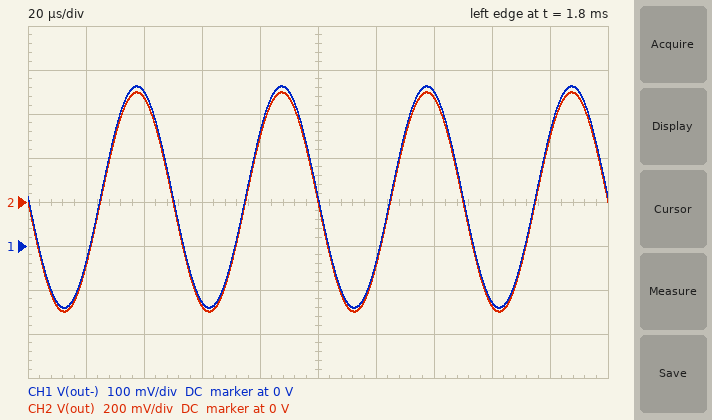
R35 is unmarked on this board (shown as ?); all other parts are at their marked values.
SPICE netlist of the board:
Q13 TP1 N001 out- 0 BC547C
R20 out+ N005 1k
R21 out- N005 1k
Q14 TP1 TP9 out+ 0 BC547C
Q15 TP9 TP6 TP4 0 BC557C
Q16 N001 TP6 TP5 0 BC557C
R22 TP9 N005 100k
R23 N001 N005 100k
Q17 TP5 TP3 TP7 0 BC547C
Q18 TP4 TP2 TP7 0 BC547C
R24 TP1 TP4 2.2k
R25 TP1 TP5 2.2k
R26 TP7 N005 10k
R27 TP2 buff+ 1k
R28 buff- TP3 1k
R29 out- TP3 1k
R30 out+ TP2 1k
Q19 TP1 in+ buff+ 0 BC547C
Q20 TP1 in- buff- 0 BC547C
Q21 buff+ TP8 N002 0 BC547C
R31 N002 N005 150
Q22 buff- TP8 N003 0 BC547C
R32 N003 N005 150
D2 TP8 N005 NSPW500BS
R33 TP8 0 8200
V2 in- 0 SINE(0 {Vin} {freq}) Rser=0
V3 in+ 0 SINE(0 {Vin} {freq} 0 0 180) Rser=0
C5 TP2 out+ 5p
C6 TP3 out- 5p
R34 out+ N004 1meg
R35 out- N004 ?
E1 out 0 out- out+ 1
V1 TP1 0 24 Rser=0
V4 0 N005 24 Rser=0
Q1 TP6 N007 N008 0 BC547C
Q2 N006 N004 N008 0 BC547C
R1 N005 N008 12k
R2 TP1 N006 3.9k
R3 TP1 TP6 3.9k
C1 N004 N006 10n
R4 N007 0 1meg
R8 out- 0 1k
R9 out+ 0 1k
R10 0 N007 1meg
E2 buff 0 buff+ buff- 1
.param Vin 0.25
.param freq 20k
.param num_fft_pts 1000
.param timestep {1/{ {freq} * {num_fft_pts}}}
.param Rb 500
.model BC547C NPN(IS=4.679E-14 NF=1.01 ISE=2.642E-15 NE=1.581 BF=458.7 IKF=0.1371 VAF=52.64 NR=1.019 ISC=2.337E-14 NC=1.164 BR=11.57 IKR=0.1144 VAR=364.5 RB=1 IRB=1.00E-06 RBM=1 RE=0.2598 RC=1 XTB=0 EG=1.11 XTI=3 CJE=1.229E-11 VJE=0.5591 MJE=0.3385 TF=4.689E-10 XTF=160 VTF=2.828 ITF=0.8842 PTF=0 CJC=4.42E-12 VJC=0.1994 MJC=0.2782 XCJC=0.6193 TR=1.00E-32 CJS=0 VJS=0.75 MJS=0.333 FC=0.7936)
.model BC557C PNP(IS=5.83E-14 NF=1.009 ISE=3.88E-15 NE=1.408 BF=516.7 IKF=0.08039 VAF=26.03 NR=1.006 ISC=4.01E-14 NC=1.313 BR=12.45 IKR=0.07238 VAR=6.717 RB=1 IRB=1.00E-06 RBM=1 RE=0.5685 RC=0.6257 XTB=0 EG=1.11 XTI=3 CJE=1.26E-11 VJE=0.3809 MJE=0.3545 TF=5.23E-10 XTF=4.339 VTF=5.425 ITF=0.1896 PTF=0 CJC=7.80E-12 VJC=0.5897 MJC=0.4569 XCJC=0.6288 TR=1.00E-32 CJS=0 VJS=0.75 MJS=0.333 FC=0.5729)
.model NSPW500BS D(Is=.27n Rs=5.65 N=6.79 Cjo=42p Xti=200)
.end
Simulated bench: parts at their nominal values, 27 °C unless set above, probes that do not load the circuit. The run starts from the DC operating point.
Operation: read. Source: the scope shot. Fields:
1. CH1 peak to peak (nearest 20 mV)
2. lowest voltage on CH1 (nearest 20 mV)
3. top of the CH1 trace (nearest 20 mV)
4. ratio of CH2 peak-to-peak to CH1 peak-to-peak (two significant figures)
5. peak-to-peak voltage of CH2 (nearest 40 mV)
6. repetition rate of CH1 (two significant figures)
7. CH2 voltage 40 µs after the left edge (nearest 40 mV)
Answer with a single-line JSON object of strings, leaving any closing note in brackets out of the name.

{"CH1 peak to peak": "500 mV", "lowest voltage on CH1": "-140 mV", "top of the CH1 trace": "360 mV", "ratio of CH2 peak-to-peak to CH1 peak-to-peak": "2.0", "peak-to-peak voltage of CH2": "1.00 V", "repetition rate of CH1": "20 kHz", "CH2 voltage 40 µs after the left edge": "480 mV"}
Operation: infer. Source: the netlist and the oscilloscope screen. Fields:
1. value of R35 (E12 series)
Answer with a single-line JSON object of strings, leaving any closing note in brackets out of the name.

{"value of R35": "1.5 MΩ"}
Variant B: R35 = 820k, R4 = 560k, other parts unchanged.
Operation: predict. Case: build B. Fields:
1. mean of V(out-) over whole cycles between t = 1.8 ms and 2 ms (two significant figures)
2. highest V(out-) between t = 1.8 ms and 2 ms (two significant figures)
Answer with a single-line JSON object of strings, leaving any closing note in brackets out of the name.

{"mean of V(out-) over whole cycles between t = 1.8 ms and 2 ms": "120 mV", "highest V(out-) between t = 1.8 ms and 2 ms": "370 mV"}
